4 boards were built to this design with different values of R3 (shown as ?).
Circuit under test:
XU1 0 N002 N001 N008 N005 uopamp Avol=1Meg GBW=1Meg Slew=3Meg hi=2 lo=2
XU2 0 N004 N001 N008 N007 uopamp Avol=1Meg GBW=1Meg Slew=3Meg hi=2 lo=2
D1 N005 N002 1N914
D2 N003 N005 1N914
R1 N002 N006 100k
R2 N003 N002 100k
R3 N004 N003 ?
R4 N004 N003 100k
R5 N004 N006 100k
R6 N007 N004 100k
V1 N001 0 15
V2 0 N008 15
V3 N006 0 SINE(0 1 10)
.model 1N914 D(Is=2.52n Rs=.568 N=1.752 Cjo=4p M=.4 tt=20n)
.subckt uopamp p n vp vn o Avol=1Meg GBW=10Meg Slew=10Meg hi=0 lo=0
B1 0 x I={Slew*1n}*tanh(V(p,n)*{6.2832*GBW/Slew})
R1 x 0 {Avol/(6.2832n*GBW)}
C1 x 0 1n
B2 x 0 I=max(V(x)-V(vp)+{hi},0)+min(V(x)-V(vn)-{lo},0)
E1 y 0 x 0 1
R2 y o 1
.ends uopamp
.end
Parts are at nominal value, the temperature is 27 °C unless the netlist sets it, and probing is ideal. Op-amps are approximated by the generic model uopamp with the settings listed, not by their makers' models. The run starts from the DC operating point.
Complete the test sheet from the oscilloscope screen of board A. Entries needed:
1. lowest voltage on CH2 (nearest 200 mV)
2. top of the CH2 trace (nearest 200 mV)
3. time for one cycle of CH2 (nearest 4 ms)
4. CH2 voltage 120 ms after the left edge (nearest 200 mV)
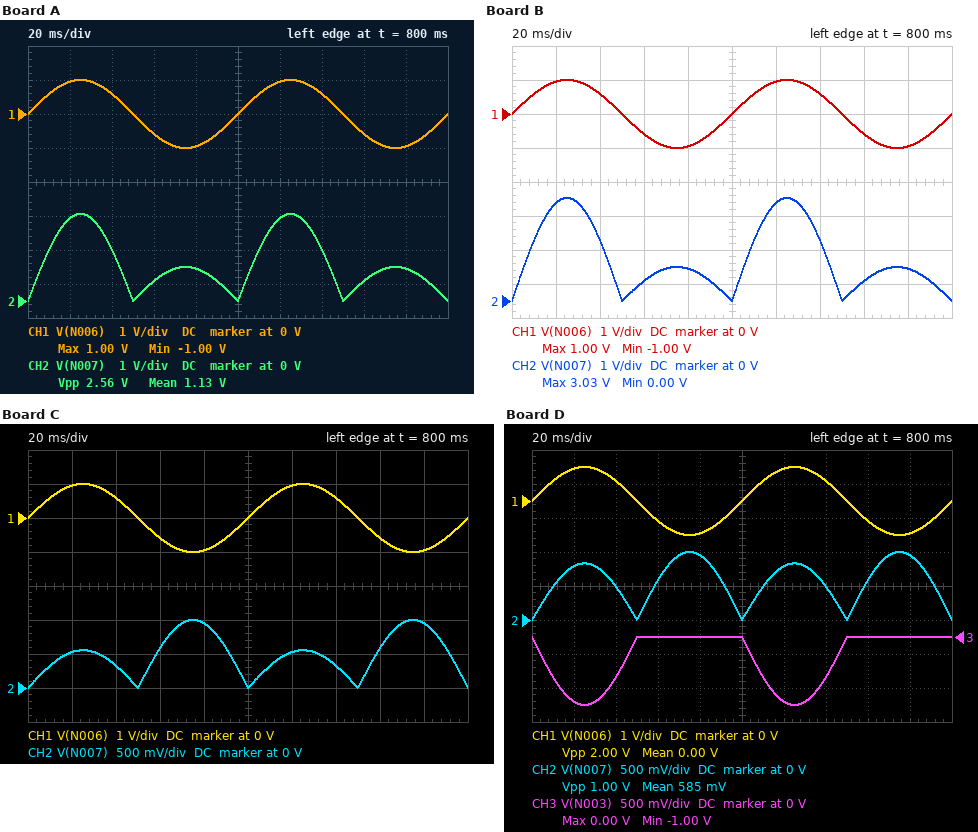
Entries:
0 V
2.6 V
100 ms
2.4 V
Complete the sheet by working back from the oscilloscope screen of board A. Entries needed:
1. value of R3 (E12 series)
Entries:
39 kΩ
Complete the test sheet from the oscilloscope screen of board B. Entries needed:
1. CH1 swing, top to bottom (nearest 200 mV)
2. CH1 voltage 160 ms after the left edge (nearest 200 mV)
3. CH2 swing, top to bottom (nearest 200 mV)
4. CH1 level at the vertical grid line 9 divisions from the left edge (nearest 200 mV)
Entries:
2.0 V
-600 mV
3.0 V
-1.0 V
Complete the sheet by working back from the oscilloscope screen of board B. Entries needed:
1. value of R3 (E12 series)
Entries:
33 kΩ
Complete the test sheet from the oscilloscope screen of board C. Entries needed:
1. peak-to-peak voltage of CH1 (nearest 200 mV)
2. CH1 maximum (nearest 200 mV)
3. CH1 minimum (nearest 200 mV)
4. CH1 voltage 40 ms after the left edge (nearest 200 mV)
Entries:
2.0 V
1.0 V
-1.0 V
600 mV
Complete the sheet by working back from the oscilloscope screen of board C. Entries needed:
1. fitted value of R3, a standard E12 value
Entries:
180 kΩ
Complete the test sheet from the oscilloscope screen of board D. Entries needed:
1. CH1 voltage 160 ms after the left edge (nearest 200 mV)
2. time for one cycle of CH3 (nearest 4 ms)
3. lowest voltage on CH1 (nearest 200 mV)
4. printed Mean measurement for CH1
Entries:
-600 mV
100 ms
-1.0 V
0.00 V
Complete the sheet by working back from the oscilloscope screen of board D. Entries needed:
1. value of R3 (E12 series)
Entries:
120 kΩ
